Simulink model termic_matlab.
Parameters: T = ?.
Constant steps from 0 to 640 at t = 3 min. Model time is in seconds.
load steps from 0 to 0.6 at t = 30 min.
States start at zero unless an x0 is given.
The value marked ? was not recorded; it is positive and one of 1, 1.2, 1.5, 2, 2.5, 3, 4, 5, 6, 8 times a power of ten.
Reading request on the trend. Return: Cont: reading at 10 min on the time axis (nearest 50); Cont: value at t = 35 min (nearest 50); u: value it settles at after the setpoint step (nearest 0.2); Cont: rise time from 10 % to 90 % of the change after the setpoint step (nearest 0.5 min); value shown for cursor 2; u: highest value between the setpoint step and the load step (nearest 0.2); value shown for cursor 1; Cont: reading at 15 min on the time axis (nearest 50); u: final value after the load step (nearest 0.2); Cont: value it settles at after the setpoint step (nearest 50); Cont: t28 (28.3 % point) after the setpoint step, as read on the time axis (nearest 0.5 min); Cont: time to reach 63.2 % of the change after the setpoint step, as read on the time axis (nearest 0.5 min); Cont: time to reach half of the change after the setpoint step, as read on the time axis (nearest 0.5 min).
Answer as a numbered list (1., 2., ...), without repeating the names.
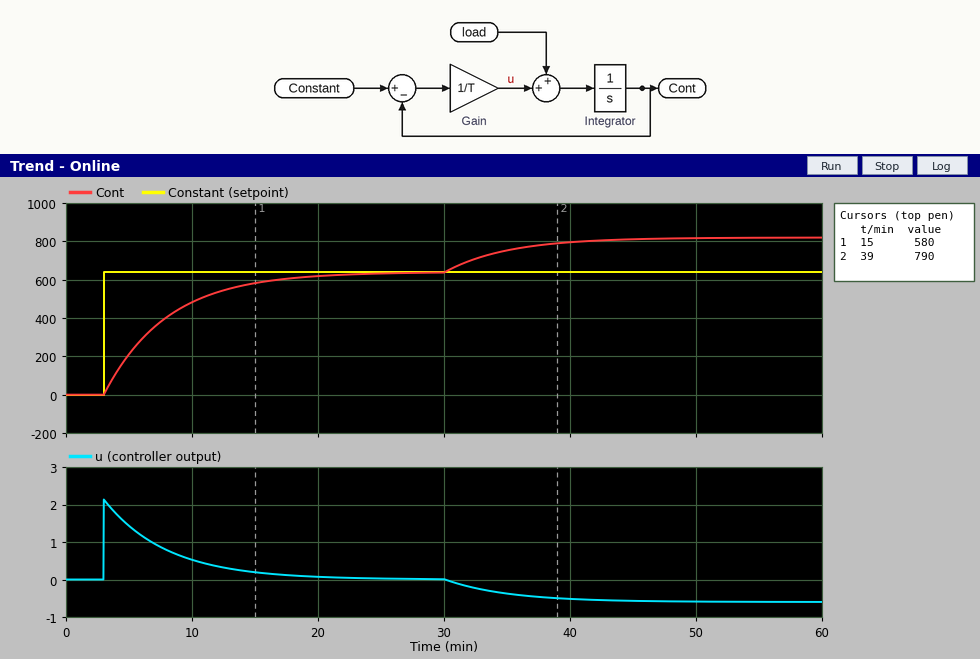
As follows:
1. 500
2. 750
3. 0.0
4. 11.0 min
5. 790
6. 2.2
7. 580
8. 600
9. -0.6
10. 650
11. 4.5 min
12. 8.0 min
13. 6.5 min
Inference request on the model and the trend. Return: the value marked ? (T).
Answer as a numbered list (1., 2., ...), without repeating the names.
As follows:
1. 300
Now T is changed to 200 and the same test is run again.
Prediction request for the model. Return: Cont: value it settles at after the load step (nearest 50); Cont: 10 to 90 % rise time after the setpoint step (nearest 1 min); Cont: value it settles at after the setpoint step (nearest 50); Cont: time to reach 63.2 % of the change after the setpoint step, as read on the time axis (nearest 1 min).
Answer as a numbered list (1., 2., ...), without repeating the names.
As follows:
1. 750
2. 7 min
3. 650
4. 6 min
